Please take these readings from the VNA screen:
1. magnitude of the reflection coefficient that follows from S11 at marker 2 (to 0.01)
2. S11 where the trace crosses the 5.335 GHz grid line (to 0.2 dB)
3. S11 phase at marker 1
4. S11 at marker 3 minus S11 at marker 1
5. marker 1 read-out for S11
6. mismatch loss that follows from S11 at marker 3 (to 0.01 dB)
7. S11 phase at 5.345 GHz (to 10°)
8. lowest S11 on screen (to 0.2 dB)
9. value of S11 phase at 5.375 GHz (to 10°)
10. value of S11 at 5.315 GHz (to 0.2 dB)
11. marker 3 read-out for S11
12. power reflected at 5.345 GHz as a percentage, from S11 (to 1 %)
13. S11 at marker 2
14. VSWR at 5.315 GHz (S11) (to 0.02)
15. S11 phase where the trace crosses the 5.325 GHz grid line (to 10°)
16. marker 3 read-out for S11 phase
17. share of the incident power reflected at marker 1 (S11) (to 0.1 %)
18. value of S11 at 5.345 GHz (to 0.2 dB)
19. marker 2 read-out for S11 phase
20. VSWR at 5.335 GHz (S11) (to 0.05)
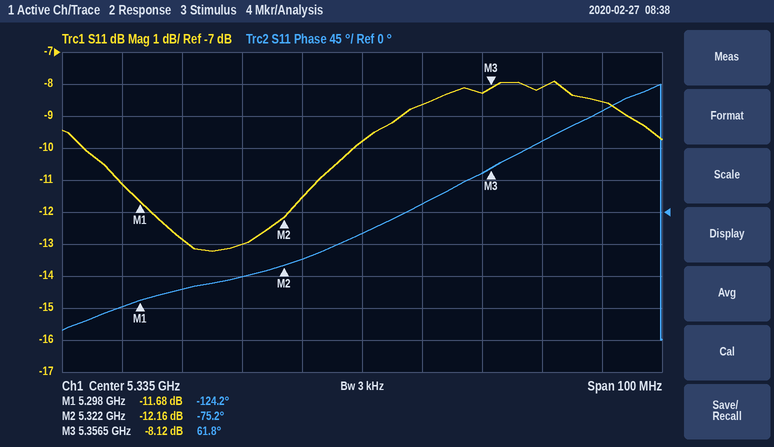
0.25
-9.8 dB
-124.2°
3.56 dB
-11.68 dB
0.73 dB
10°
-13.2 dB
140°
-13.0 dB
-8.12 dB
14 %
-12.16 dB
1.58
-70°
61.8°
6.8 %
-8.6 dB
-75.2°
1.95
